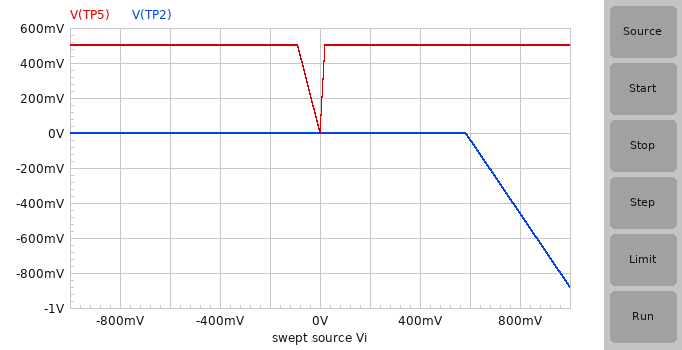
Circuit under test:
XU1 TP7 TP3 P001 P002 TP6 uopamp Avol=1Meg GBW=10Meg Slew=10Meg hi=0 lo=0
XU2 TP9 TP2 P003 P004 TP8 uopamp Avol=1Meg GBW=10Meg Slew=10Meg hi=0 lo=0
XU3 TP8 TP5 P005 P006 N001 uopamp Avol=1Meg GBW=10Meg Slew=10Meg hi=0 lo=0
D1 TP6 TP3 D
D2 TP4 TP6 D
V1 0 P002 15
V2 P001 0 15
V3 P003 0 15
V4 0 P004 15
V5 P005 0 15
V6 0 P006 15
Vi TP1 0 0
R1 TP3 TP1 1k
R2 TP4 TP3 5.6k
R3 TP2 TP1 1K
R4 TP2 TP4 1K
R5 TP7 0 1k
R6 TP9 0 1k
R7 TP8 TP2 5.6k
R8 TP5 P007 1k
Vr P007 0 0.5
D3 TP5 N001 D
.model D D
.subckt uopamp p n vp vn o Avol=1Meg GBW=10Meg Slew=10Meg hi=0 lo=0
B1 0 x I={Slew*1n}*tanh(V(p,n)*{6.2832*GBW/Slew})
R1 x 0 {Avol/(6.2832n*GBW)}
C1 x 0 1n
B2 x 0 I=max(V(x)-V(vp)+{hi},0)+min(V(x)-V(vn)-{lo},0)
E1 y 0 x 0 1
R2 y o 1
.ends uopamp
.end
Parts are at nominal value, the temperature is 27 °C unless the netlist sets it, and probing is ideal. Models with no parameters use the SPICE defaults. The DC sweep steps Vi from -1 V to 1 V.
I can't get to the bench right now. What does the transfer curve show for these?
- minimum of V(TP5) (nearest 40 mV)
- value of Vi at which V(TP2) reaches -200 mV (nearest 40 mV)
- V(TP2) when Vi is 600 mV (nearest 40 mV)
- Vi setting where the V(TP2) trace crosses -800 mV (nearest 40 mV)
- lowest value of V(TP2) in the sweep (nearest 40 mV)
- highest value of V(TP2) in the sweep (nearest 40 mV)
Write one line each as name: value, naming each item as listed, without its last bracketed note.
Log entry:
minimum of V(TP5): 0 V
value of Vi at which V(TP2) reaches -200 mV: 680 mV
V(TP2) when Vi is 600 mV: -40 mV
Vi setting where the V(TP2) trace crosses -800 mV: 960 mV
lowest value of V(TP2) in the sweep: -880 mV
highest value of V(TP2) in the sweep: 0 V
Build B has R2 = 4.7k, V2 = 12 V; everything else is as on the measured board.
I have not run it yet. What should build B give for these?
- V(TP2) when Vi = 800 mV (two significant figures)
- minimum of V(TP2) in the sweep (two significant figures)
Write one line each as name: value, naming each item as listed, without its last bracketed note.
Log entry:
V(TP2) when Vi = 800 mV: -130 mV
minimum of V(TP2) in the sweep: -470 mV
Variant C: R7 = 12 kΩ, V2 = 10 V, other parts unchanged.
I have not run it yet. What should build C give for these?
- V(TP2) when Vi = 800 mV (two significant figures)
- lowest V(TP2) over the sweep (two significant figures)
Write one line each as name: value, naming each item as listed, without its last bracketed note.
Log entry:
V(TP2) when Vi = 800 mV: -1.2 V
lowest V(TP2) over the sweep: -1.6 V
